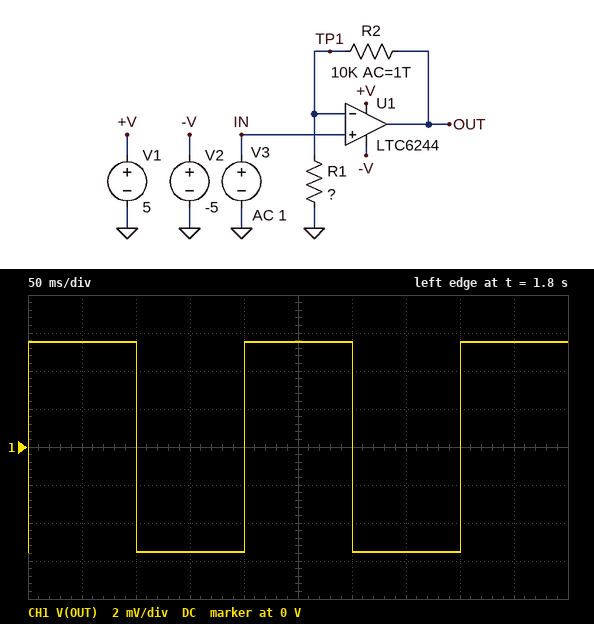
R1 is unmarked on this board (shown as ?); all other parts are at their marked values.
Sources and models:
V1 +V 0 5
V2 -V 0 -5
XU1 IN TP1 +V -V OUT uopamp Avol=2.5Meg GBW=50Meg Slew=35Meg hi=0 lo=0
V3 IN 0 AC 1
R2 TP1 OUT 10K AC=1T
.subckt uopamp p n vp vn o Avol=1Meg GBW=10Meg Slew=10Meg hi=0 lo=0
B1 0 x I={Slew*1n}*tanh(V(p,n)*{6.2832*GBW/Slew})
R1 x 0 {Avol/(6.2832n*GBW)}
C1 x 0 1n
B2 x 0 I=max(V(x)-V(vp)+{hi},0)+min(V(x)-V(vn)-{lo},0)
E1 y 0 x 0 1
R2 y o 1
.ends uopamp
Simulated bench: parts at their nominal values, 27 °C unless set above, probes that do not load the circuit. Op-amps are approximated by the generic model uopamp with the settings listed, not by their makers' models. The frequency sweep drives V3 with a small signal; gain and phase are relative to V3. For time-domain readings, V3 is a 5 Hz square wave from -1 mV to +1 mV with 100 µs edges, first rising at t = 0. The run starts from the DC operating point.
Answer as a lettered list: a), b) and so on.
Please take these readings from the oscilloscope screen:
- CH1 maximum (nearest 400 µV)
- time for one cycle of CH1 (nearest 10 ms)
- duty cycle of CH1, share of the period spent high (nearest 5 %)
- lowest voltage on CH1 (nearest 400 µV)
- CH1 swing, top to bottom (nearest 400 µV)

a) 5.6 mV
b) 200 ms
c) 50 %
d) -5.6 mV
e) 11.2 mV
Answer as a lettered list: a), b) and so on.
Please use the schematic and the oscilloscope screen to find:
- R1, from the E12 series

a) 2.2 kΩ
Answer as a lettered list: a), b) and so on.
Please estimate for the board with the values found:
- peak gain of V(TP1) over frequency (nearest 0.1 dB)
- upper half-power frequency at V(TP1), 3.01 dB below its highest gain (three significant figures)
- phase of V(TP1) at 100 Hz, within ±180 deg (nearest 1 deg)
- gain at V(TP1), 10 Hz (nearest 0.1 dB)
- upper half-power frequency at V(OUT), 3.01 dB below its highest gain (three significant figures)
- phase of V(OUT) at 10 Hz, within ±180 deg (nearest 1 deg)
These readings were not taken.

a) -45.2 dB
b) 20.1 Hz
c) -79 deg
d) -46.2 dB
e) 20.1 Hz
f) -26 deg
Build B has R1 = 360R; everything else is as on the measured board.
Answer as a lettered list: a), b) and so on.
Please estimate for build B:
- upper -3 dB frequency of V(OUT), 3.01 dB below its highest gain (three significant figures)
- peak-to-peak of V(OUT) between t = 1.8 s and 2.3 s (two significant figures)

a) 20.0 Hz
b) 58 mV
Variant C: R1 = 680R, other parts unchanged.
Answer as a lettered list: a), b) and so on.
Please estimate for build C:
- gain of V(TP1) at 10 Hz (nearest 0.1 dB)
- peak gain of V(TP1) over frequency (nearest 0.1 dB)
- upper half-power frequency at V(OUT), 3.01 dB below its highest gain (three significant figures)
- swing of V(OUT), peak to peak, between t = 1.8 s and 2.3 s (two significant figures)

a) -56.4 dB
b) -55.4 dB
c) 20.0 Hz
d) 31 mV
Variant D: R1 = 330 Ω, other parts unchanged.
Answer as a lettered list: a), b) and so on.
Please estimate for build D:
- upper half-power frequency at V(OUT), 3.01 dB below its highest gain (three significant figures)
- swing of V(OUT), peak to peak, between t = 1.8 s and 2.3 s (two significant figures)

a) 20.0 Hz
b) 63 mV
